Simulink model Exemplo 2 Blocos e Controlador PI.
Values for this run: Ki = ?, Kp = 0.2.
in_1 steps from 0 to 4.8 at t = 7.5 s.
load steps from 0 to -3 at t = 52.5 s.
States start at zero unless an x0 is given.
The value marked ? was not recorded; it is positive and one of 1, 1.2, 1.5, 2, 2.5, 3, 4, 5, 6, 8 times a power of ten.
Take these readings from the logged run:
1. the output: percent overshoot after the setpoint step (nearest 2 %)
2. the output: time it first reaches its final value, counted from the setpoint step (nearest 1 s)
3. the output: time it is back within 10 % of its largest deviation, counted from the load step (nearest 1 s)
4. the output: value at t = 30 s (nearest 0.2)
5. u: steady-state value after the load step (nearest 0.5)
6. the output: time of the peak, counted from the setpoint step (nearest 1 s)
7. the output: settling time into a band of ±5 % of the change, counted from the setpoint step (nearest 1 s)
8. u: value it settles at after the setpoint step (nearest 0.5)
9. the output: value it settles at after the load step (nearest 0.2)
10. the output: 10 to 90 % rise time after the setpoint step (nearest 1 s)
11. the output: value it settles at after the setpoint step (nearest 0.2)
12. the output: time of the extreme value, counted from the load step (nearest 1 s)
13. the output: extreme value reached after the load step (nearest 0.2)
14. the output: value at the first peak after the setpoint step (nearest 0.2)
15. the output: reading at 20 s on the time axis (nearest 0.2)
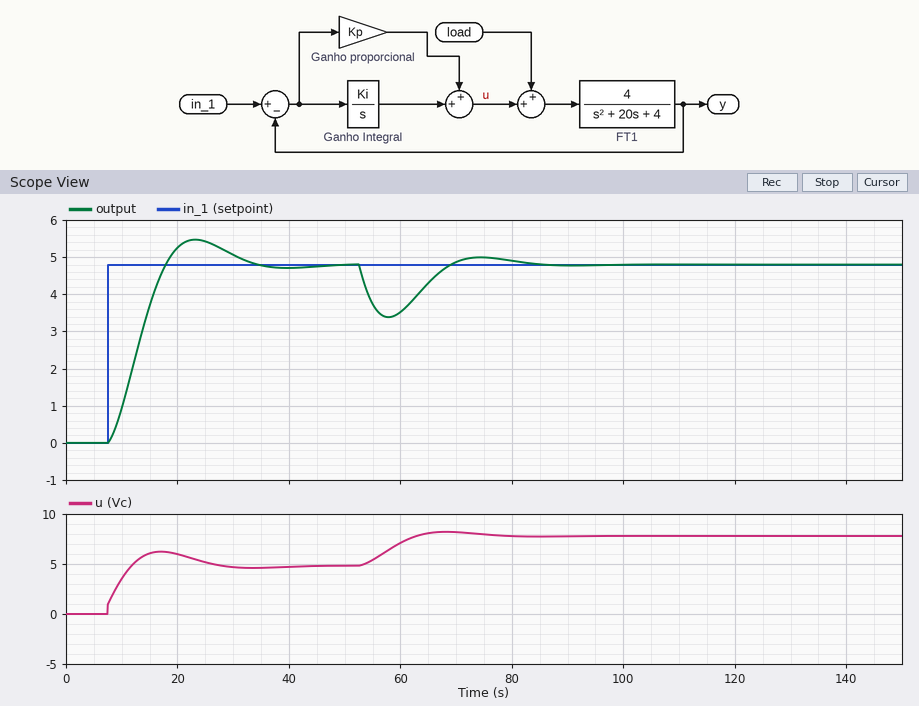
14 %
10 s
26 s
5.0
8.0
16 s
23 s
5.0
4.8
7 s
4.8
5 s
3.4
5.4
5.2
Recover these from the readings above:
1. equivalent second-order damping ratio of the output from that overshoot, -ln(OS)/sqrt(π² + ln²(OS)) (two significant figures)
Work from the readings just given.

0.53
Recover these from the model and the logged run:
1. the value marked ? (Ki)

0.25
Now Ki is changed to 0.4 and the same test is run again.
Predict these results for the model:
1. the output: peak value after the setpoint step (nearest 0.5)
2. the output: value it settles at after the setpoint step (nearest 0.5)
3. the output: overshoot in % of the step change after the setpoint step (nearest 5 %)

6.0
5.0
25 %
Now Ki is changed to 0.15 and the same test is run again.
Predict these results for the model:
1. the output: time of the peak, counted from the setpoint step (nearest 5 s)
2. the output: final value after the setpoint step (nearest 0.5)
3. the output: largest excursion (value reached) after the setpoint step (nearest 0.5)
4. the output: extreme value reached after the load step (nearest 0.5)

25 s
5.0
5.0
3.0
